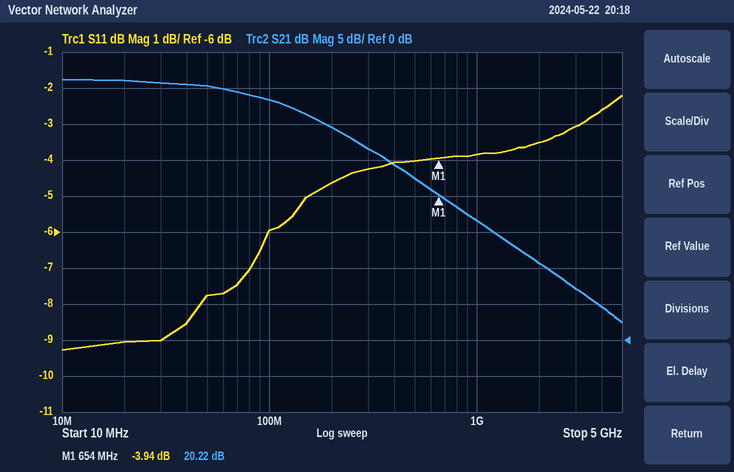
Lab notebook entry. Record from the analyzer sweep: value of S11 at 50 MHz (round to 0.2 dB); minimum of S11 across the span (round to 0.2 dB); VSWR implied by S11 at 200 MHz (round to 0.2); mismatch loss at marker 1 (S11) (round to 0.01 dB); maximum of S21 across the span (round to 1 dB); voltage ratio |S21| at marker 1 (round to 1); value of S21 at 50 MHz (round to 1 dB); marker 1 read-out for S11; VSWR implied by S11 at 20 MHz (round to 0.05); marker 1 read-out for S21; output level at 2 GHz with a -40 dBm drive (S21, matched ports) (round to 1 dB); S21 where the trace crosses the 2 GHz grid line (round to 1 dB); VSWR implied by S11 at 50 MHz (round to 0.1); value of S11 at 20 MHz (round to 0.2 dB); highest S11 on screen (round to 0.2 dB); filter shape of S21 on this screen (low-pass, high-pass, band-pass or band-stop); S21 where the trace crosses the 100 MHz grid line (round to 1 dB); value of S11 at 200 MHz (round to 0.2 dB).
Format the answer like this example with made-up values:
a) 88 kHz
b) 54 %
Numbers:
a) -7.8 dB
b) -9.2 dB
c) 3.8
d) 2.24 dB
e) 36 dB
f) 10
g) 35 dB
h) -3.94 dB
i) 2.10
j) 20.22 dB
k) -29 dBm
l) 11 dB
m) 2.4
n) -9.0 dB
o) -2.2 dB
p) low-pass
q) 33 dB
r) -4.6 dB
